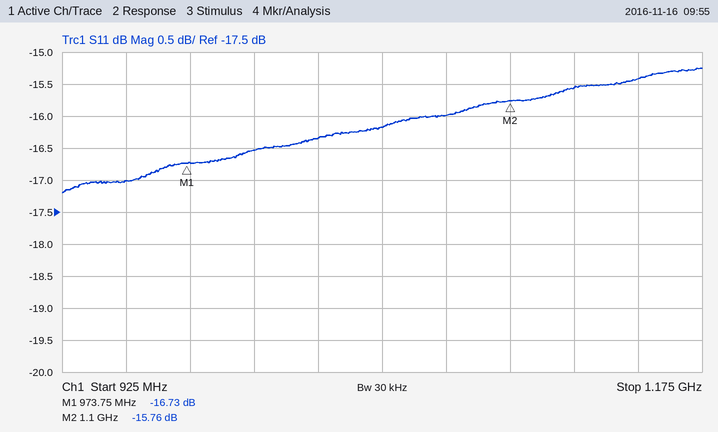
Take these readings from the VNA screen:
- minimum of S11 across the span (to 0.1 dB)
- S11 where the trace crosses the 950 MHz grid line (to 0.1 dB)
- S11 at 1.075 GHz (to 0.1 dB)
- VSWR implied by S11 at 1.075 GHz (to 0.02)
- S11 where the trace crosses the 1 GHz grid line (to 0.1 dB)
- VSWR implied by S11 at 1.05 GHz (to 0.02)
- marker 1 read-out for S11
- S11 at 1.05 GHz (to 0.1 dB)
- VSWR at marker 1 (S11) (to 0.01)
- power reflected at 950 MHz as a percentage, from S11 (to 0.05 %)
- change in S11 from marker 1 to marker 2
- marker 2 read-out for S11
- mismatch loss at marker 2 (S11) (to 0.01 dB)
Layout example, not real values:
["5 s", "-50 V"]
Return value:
["-17.2 dB", "-17.0 dB", "-16.0 dB", "1.38", "-16.5 dB", "1.36", "-16.73 dB", "-16.2 dB", "1.34", "2.00 %", "0.97 dB", "-15.76 dB", "0.12 dB"]
